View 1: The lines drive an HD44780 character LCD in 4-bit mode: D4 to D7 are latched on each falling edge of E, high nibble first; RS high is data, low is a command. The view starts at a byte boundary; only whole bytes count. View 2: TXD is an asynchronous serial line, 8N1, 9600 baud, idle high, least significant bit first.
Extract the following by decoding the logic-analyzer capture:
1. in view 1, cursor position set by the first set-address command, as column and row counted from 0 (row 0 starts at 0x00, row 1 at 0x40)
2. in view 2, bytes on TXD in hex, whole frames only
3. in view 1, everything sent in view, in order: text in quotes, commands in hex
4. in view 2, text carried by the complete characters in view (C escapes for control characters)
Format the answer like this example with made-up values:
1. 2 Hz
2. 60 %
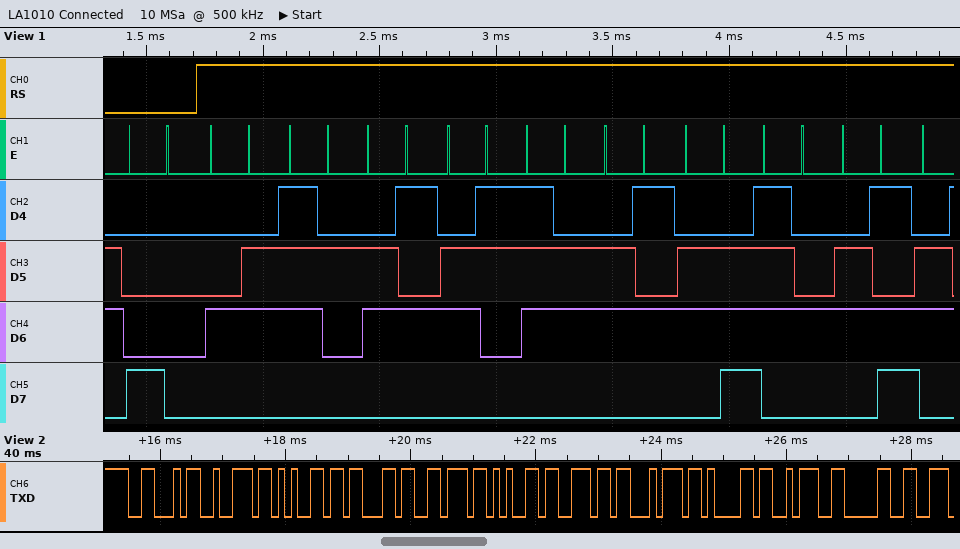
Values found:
1. column 0, row 0
2. 46 72 65 63 76 65 6E 74 61 3A 30
3. 0x80 "Frecventm"
4. "Frecventa:0"
